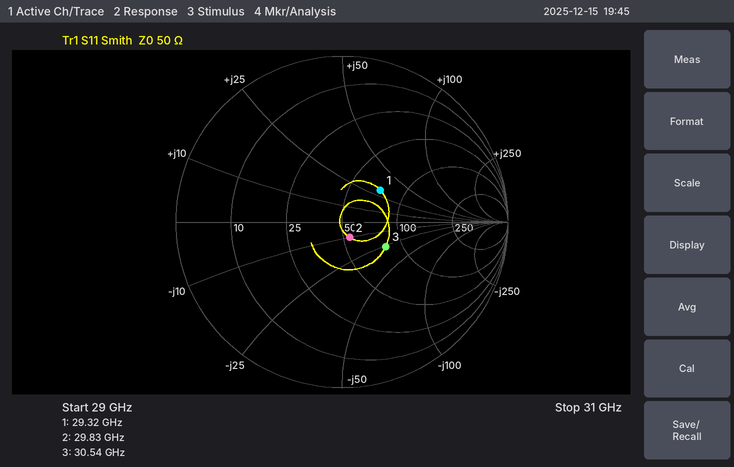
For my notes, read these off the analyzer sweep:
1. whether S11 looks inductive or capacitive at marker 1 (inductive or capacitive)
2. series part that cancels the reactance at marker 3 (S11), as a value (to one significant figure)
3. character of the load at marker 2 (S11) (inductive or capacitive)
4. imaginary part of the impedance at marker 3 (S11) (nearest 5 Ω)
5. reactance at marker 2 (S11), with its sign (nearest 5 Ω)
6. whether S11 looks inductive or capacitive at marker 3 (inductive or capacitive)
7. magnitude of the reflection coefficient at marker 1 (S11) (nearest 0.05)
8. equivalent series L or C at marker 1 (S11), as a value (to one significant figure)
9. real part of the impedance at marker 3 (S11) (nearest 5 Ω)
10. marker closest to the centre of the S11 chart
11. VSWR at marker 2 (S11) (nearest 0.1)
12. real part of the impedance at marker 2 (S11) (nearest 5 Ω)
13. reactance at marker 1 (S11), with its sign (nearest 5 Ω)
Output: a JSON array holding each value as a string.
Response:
["inductive", "100 pH", "capacitive", "-25 Ω", "-10 Ω", "capacitive", "0.30", "200 pH", "80 Ω", "marker 2", "1.2", "55 Ω", "+30 Ω"]
